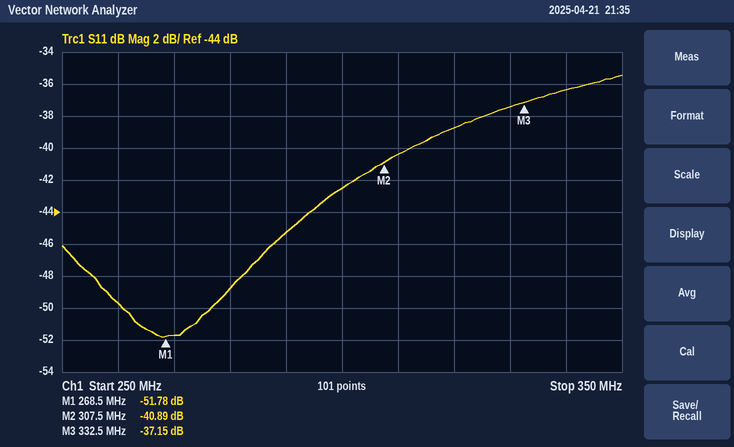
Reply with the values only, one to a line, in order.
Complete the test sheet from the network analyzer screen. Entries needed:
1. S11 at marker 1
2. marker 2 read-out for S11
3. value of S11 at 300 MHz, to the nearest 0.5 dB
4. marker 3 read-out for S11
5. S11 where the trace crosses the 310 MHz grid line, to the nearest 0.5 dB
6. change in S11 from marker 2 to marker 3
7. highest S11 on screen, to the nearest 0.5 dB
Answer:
-51.78 dB
-40.89 dB
-42.5 dB
-37.15 dB
-40.5 dB
3.74 dB
-35.5 dB
